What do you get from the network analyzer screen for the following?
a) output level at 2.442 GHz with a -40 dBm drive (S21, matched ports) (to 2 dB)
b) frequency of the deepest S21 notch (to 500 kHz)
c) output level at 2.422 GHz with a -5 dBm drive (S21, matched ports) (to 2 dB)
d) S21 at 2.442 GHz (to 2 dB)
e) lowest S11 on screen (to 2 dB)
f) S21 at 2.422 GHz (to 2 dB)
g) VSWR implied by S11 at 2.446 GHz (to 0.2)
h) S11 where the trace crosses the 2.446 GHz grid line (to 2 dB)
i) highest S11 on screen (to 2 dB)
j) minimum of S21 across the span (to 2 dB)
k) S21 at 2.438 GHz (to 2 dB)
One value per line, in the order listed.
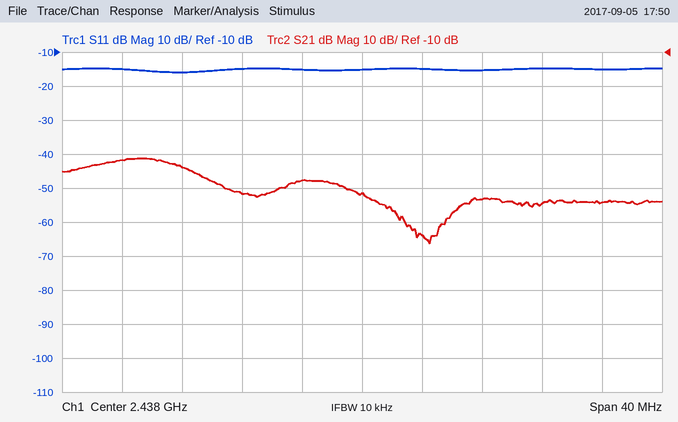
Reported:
-104 dBm
2.4425 GHz
-46 dBm
-64 dB
-16 dB
-42 dB
1.4
-16 dB
-14 dB
-66 dB
-52 dB
